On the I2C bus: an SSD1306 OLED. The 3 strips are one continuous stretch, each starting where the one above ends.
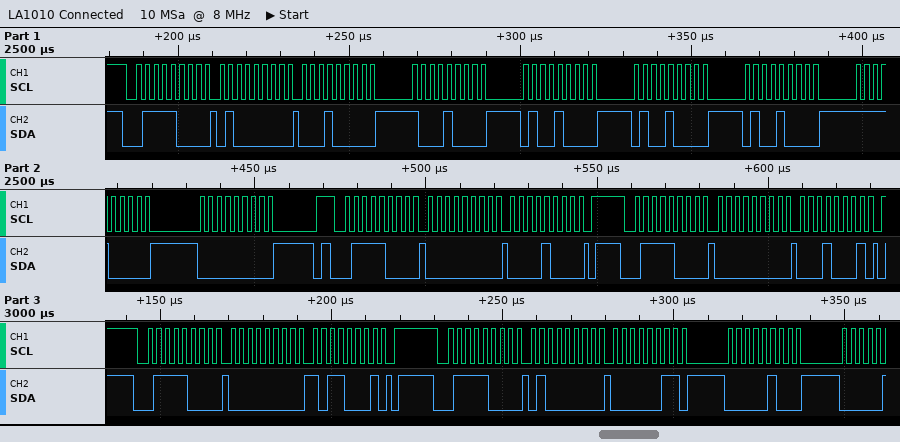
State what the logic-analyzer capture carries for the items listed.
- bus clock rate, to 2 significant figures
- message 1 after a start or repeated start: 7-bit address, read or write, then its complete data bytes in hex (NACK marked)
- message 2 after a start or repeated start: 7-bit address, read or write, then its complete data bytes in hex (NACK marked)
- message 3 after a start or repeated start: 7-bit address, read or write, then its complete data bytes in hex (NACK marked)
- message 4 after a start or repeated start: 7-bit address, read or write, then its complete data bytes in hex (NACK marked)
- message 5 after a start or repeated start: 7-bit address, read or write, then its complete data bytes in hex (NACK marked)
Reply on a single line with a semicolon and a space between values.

400 kHz; 0x3C write: 40 10 88 48 48 48 F0 00; 0x3C write: 00 08; 0x3C write: 00 11; 0x3C write: 00 B1; 0x3C write: 40 03 04
